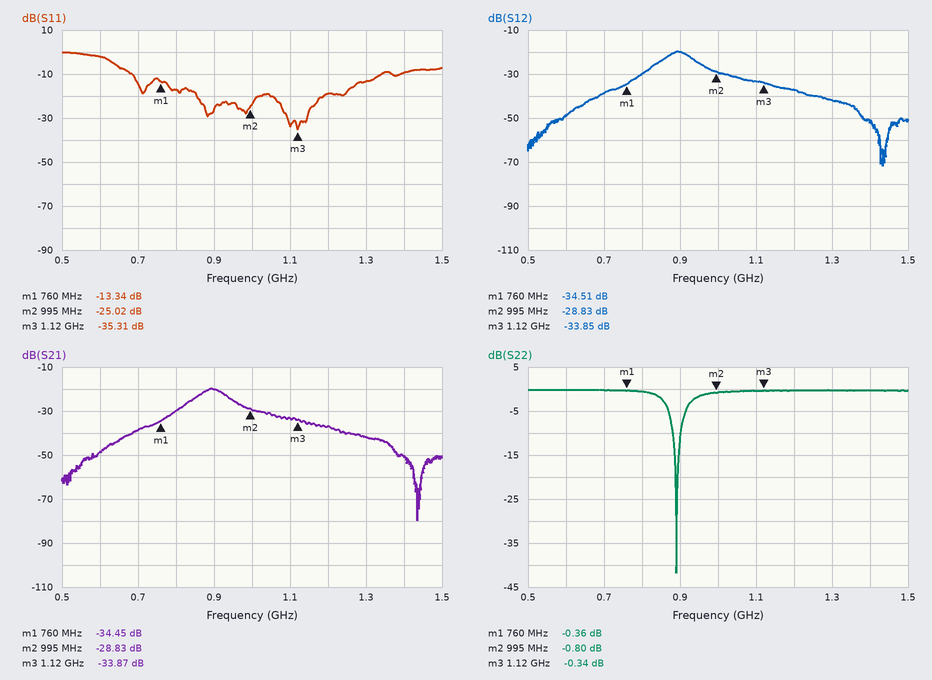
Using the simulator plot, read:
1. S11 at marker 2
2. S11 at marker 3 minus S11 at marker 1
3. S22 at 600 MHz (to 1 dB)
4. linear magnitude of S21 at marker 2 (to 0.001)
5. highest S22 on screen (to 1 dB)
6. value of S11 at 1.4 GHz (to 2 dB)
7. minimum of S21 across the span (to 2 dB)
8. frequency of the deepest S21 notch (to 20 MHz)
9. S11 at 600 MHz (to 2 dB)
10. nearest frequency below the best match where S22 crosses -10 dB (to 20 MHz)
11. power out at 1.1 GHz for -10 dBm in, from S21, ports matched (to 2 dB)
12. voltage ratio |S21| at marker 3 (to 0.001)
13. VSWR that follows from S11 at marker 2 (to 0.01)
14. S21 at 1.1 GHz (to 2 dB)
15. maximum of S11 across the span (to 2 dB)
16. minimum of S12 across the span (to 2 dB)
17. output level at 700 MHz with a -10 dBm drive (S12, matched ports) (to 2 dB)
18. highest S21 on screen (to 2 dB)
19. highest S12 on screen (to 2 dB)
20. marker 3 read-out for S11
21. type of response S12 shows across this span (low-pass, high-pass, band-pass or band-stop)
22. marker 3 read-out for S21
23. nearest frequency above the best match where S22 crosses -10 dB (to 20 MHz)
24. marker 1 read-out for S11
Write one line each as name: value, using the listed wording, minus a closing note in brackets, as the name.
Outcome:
S11 at marker 2: -25.02 dB
S11 at marker 3 minus S11 at marker 1: -21.97 dB
S22 at 600 MHz: 0 dB
linear magnitude of S21 at marker 2: 0.036
highest S22 on screen: 0 dB
value of S11 at 1.4 GHz: -10 dB
minimum of S21 across the span: -80 dB
frequency of the deepest S21 notch: 1.44 GHz
S11 at 600 MHz: -2 dB
nearest frequency below the best match where S22 crosses -10 dB: 880 MHz
power out at 1.1 GHz for -10 dBm in, from S21, ports matched: -44 dBm
voltage ratio |S21| at marker 3: 0.020
VSWR that follows from S11 at marker 2: 1.12
S21 at 1.1 GHz: -34 dB
maximum of S11 across the span: 0 dB
minimum of S12 across the span: -72 dB
output level at 700 MHz with a -10 dBm drive (S12, matched ports): -48 dBm
highest S21 on screen: -20 dB
highest S12 on screen: -20 dB
marker 3 read-out for S11: -35.31 dB
type of response S12 shows across this span: band-pass
marker 3 read-out for S21: -33.87 dB
nearest frequency above the best match where S22 crosses -10 dB: 900 MHz
marker 1 read-out for S11: -13.34 dB
